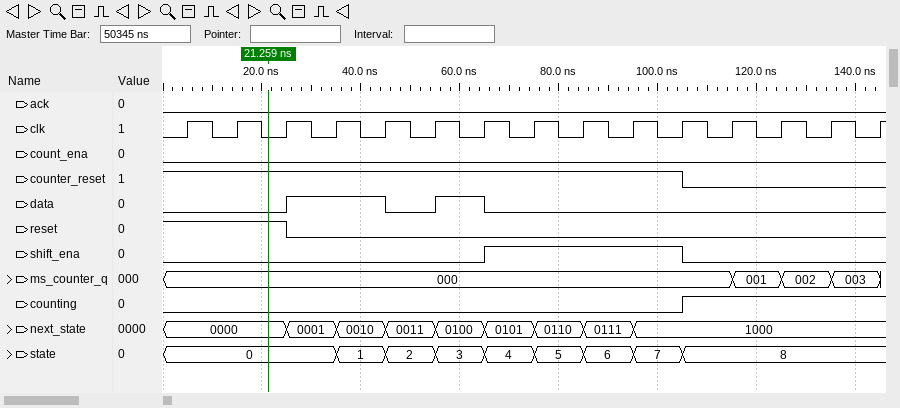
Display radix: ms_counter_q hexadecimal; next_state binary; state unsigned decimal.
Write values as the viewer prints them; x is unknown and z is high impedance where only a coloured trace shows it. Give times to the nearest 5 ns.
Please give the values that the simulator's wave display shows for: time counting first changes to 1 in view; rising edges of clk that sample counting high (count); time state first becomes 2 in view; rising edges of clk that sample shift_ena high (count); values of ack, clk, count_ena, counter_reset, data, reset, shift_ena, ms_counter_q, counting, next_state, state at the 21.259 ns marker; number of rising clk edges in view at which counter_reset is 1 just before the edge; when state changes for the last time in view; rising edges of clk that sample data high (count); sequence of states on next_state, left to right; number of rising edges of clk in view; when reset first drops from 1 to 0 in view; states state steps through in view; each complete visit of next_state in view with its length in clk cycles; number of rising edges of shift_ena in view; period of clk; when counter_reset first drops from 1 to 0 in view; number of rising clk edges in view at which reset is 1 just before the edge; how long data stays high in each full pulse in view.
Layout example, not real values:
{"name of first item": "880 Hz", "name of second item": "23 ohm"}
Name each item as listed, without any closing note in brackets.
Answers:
{"time counting first changes to 1 in view": "105 ns", "rising edges of clk that sample counting high": "4", "time state first becomes 2 in view": "45 ns", "rising edges of clk that sample shift_ena high": "4", "values of ack, clk, count_ena, counter_reset, data, reset, shift_ena, ms_counter_q, counting, next_state, state at the 21.259 ns marker": "ack=0, clk=0, count_ena=0, counter_reset=1, data=0, reset=1, shift_ena=0, ms_counter_q=000, counting=0, next_state=0000, state=0", "number of rising clk edges in view at which counter_reset is 1 just before the edge": "11", "when state changes for the last time in view": "105 ns", "rising edges of clk that sample data high": "3", "sequence of states on next_state, left to right": "0000, 0001, 0010, 0011, 0100, 0101, 0110, 0111, 1000", "number of rising edges of clk in view": "15", "when reset first drops from 1 to 0 in view": "25 ns", "states state steps through in view": "0, 1, 2, 3, 4, 5, 6, 7, 8", "each complete visit of next_state in view with its length in clk cycles": "0001: 1, 0010: 1, 0011: 1, 0100: 1, 0101: 1, 0110: 1, 0111: 1", "number of rising edges of shift_ena in view": "1", "period of clk": "10 ns", "when counter_reset first drops from 1 to 0 in view": "105 ns", "number of rising clk edges in view at which reset is 1 just before the edge": "3", "how long data stays high in each full pulse in view": "20 ns, 10 ns"}
